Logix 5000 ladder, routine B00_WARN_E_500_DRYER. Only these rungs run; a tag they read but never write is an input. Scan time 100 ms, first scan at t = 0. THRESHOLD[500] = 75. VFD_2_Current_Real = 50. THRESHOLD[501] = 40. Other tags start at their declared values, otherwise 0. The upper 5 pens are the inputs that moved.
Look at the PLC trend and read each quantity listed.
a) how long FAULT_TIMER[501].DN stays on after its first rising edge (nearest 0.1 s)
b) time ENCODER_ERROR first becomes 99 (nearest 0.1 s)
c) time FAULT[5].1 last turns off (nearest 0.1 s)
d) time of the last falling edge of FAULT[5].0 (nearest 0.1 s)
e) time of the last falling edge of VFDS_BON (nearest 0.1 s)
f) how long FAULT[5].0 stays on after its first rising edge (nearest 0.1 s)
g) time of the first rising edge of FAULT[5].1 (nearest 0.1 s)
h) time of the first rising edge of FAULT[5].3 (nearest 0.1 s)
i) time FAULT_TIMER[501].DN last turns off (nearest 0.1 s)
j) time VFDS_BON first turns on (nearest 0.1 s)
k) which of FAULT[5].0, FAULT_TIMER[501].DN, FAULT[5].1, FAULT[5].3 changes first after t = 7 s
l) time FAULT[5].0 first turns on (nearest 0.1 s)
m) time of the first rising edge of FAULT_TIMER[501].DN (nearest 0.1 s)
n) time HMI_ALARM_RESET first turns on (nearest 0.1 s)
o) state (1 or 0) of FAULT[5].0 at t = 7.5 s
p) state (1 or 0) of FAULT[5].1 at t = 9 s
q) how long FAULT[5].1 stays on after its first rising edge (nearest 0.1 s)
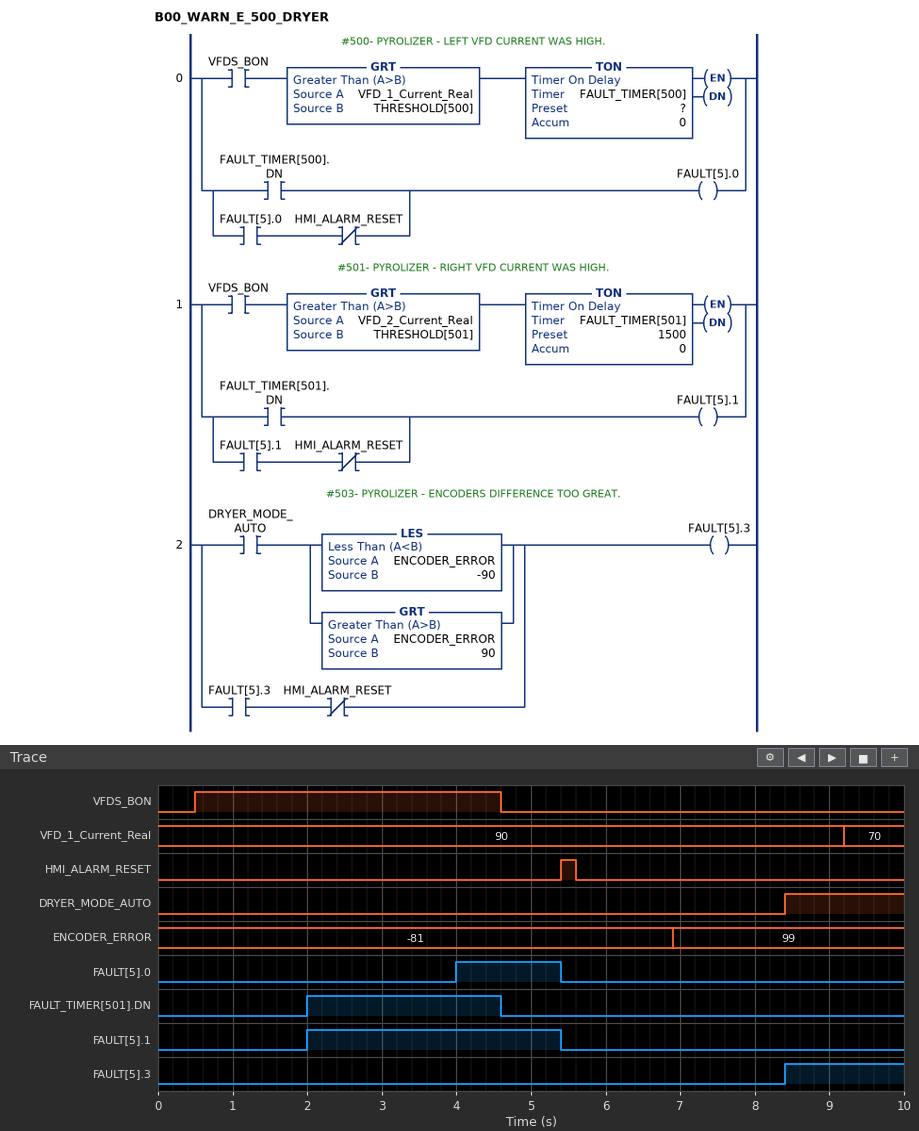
2.6 s
6.9 s
5.4 s
5.4 s
4.6 s
1.4 s
2.0 s
8.4 s
4.6 s
0.5 s
FAULT[5].3
4.0 s
2.0 s
5.4 s
0
0
3.4 s
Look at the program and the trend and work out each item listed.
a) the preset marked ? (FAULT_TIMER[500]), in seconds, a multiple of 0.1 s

3.5 s
